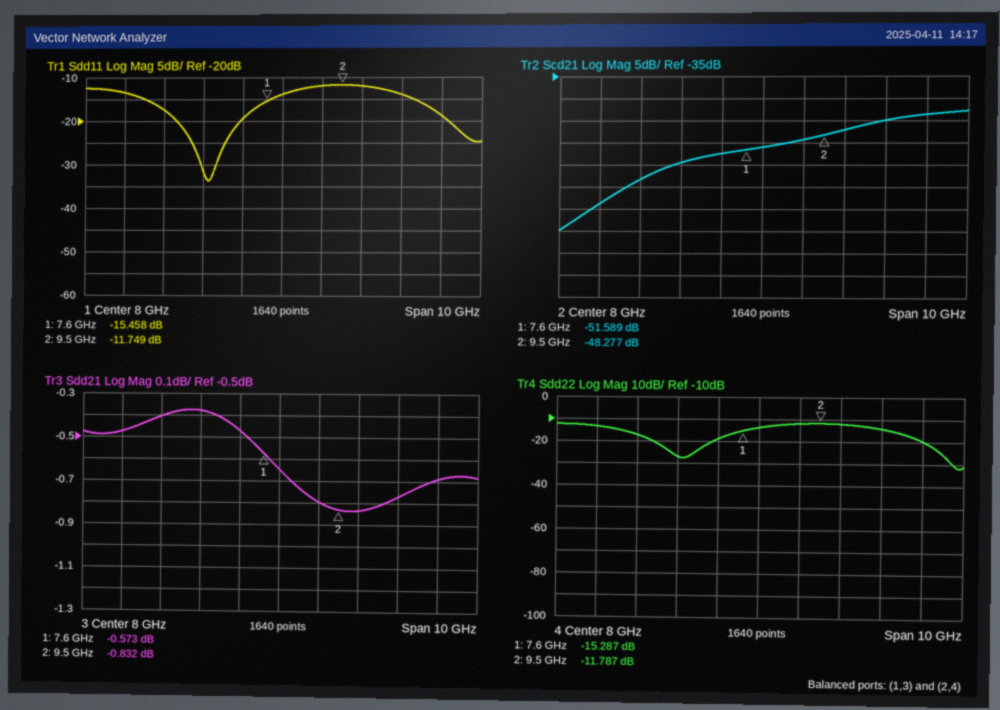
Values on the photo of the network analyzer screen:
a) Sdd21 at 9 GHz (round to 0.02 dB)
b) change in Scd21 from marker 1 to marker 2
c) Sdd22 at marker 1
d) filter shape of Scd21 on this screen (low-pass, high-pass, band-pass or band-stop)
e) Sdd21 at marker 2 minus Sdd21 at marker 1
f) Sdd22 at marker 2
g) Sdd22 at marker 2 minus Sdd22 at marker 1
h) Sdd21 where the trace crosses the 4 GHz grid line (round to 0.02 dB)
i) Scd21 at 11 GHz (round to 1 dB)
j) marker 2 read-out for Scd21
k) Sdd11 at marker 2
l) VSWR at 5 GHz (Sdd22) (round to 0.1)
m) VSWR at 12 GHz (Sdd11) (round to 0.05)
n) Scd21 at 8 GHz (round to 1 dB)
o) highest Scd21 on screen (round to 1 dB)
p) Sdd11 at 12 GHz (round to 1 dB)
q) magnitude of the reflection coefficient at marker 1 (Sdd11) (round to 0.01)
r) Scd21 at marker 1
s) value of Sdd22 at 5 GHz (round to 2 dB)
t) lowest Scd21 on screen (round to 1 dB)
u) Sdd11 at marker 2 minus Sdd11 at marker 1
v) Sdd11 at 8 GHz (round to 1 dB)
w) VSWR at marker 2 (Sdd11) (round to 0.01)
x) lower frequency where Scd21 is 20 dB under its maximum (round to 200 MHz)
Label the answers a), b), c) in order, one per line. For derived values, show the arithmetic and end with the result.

a) -0.80 dB
b) -48.277 − (-51.589) = 3.312 dB
c) -15.287 dB
d) high-pass
e) -0.832 − (-0.573) = -0.259 dB
f) -11.787 dB
g) -11.787 − (-15.287) = 3.500 dB
h) -0.48 dB
i) -45 dB
j) -48.277 dB
k) -11.749 dB
l) |Γ| = 10^(-18/20) = 0.1259; VSWR = (1 + 0.1259)/(1 − 0.1259) ≈ 1.3
m) |Γ| = 10^(-19/20) = 0.1122; VSWR = (1 + 0.1122)/(1 − 0.1122) ≈ 1.25
n) -51 dB
o) -43 dB
p) -19 dB
q) 10^(-15.458/20) ≈ 0.17
r) -51.589 dB
s) -18 dB
t) -70 dB
u) -11.749 − (-15.458) = 3.709 dB
v) -14 dB
w) (1 + 0.2586)/(1 − 0.2586) ≈ 1.70
x) 4.2 GHz
